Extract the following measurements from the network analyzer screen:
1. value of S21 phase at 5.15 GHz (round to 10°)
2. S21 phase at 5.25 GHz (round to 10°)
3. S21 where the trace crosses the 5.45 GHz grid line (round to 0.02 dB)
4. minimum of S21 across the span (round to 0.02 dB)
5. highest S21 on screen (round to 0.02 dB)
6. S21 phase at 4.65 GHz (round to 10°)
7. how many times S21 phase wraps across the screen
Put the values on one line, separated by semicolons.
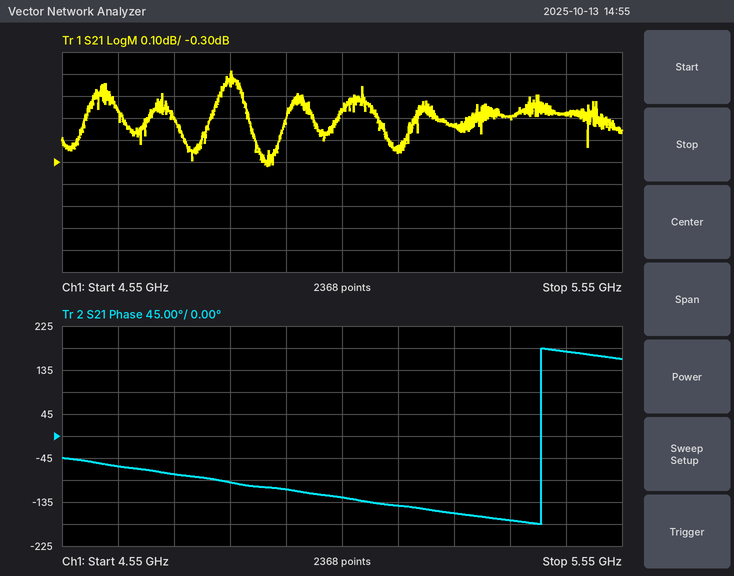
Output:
-140°; -160°; -0.08 dB; -0.32 dB; 0.12 dB; -60°; 1
